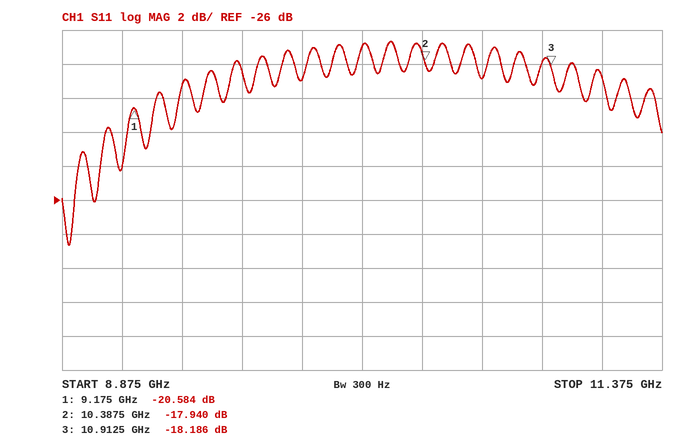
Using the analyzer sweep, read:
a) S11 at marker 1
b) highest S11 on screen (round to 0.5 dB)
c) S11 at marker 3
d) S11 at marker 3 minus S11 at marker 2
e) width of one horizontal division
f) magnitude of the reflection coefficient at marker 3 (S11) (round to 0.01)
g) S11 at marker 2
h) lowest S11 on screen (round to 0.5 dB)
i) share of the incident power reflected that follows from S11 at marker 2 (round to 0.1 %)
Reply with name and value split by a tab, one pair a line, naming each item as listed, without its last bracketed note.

S11 at marker 1	-20.584 dB
highest S11 on screen	-16.5 dB
S11 at marker 3	-18.186 dB
S11 at marker 3 minus S11 at marker 2	-0.246 dB
width of one horizontal division	250 MHz
magnitude of the reflection coefficient at marker 3 (S11)	0.12
S11 at marker 2	-17.940 dB
lowest S11 on screen	-28.5 dB
share of the incident power reflected that follows from S11 at marker 2	1.6 %
